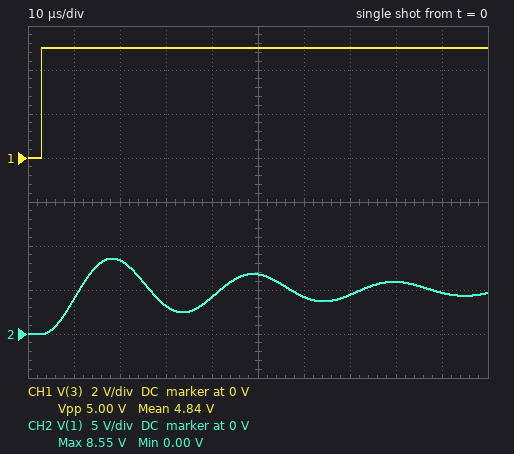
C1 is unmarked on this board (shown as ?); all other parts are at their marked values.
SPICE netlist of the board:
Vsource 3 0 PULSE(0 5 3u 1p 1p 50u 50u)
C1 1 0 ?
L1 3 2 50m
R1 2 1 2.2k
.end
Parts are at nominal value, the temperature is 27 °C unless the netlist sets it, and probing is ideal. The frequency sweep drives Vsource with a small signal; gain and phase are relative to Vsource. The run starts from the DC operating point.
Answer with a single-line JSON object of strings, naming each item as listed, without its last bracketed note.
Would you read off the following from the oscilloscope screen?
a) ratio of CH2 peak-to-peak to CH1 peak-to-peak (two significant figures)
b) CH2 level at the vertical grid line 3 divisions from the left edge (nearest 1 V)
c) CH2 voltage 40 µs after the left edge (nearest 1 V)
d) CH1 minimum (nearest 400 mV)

{"ratio of CH2 peak-to-peak to CH1 peak-to-peak": "1.7", "CH2 level at the vertical grid line 3 divisions from the left edge": "3 V", "CH2 voltage 40 µs after the left edge": "4 V", "CH1 minimum": "0 V"}
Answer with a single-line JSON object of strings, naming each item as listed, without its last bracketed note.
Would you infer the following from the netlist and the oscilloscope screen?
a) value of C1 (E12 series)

{"value of C1": "470 pF"}
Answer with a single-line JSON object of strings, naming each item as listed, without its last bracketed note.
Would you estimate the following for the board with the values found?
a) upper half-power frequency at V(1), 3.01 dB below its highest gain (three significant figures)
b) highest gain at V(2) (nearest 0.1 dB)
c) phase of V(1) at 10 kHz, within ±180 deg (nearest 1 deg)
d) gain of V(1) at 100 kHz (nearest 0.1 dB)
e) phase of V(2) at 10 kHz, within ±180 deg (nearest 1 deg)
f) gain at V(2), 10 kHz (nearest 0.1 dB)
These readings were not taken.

{"upper half-power frequency at V(1), 3.01 dB below its highest gain": "35.8 kHz", "highest gain at V(2)": "13.7 dB", "phase of V(1) at 10 kHz, within ±180 deg": "-4 deg", "gain of V(1) at 100 kHz": "-18.4 dB", "phase of V(2) at 10 kHz, within ±180 deg": "0 deg", "gain at V(2), 10 kHz": "0.8 dB"}
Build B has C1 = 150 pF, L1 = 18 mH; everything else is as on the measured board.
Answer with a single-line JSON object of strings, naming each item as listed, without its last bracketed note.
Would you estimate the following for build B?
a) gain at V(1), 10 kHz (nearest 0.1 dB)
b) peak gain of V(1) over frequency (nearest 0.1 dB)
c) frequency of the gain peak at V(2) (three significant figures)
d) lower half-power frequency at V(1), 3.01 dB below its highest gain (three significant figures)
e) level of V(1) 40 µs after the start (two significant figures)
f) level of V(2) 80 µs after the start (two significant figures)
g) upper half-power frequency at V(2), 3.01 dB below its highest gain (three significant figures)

{"gain at V(1), 10 kHz": "0.1 dB", "peak gain of V(1) over frequency": "14.0 dB", "frequency of the gain peak at V(2)": "95.9 kHz", "lower half-power frequency at V(1), 3.01 dB below its highest gain": "85.5 kHz", "level of V(1) 40 µs after the start": "5.5 V", "level of V(2) 80 µs after the start": "5.0 V", "upper half-power frequency at V(2), 3.01 dB below its highest gain": "105 kHz"}
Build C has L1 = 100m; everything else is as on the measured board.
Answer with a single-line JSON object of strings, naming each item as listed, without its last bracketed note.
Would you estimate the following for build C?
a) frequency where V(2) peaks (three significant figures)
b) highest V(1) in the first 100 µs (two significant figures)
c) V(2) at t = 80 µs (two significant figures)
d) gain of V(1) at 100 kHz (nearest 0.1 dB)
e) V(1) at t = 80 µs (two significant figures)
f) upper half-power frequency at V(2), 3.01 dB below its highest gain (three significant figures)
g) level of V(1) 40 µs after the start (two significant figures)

{"frequency where V(2) peaks": "23.1 kHz", "highest V(1) in the first 100 µs": "8.9 V", "V(2) at t = 80 µs": "4.4 V", "gain of V(1) at 100 kHz": "-24.9 dB", "V(1) at t = 80 µs": "4.7 V", "upper half-power frequency at V(2), 3.01 dB below its highest gain": "24.8 kHz", "level of V(1) 40 µs after the start": "3.1 V"}
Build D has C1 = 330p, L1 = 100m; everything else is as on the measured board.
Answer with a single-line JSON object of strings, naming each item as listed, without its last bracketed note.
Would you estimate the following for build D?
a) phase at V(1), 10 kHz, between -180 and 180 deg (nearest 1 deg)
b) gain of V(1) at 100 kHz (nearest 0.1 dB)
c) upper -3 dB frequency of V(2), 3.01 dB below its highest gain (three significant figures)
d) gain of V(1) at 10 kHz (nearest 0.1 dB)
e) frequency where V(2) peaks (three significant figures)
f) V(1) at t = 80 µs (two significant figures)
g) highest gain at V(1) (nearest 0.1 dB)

{"phase at V(1), 10 kHz, between -180 and 180 deg": "-3 deg", "gain of V(1) at 100 kHz": "-21.6 dB", "upper -3 dB frequency of V(2), 3.01 dB below its highest gain": "29.3 kHz", "gain of V(1) at 10 kHz": "1.2 dB", "frequency where V(2) peaks": "27.6 kHz", "V(1) at t = 80 µs": "3.4 V", "highest gain at V(1)": "18.0 dB"}
